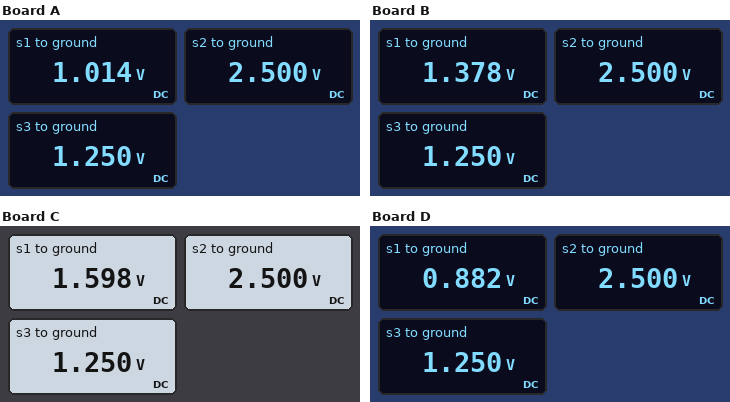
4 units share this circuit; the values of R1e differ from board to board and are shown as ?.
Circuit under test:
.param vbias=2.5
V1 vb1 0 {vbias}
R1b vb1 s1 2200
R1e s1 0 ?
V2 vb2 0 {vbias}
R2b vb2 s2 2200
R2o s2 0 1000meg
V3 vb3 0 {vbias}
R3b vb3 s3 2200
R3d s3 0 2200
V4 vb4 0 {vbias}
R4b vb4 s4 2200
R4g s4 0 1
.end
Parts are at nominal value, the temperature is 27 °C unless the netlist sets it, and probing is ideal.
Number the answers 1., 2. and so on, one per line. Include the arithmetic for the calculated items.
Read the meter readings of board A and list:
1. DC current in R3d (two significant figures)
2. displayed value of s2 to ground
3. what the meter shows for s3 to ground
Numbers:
1. (1.25 V) / 2.2 kΩ = 570 µA
2. 2.500 V
3. 1.250 V
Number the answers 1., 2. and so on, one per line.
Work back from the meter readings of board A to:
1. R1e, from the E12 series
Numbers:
1. 1.5 kΩ
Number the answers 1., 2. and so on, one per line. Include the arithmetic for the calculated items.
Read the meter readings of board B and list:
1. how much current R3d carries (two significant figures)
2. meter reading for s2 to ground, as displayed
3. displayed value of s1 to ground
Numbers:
1. (1.25 V) / 2.2 kΩ = 570 µA
2. 2.500 V
3. 1.378 V
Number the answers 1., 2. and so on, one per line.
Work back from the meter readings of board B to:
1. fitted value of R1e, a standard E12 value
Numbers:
1. 2.7 kΩ
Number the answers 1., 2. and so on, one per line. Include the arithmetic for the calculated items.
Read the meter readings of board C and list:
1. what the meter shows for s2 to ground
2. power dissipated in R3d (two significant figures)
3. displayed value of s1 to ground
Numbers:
1. 2.500 V
2. (1.25 V)^2 / 2.2 kΩ = 710 µW
3. 1.598 V
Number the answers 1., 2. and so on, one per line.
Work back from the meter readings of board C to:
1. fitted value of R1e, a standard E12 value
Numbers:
1. 3.9 kΩ
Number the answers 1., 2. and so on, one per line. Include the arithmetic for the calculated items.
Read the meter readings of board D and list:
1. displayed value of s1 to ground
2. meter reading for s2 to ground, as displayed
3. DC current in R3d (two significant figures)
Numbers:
1. 0.882 V
2. 2.500 V
3. (1.25 V) / 2.2 kΩ = 570 µA
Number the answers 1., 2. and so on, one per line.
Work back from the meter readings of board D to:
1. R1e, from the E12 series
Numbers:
1. 1.2 kΩ
